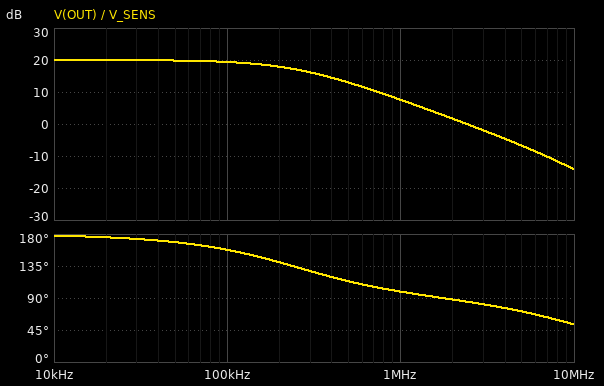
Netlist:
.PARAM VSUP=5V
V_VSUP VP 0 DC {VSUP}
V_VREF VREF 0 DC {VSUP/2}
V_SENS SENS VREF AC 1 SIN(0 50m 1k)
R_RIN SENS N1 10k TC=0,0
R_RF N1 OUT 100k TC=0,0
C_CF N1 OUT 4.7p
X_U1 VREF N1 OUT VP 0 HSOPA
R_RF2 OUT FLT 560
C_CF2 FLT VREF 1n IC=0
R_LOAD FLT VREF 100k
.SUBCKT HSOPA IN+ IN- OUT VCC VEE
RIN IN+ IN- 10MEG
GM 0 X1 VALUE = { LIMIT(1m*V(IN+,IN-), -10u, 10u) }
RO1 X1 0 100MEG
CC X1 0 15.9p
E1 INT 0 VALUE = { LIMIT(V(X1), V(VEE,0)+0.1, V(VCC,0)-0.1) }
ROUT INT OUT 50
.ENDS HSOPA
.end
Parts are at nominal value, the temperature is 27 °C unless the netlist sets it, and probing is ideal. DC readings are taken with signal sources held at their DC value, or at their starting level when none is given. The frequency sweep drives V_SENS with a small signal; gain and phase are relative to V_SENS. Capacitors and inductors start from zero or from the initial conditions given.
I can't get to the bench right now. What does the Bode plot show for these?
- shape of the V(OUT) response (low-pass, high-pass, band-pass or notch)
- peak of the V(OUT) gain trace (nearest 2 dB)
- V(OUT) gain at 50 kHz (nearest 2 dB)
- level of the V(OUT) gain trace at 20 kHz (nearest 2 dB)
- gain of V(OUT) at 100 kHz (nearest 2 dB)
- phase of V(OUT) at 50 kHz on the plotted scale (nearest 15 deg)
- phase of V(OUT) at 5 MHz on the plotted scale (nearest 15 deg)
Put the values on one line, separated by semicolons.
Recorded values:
low-pass; 20 dB; 20 dB; 20 dB; 20 dB; 165 deg; 75 deg
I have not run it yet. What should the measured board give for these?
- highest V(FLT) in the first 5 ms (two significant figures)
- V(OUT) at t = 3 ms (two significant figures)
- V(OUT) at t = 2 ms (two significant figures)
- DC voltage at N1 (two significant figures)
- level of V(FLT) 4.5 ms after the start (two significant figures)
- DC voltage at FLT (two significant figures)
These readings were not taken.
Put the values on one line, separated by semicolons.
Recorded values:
3.0 V; 2.5 V; 2.5 V; 2.5 V; 2.5 V; 2.5 V
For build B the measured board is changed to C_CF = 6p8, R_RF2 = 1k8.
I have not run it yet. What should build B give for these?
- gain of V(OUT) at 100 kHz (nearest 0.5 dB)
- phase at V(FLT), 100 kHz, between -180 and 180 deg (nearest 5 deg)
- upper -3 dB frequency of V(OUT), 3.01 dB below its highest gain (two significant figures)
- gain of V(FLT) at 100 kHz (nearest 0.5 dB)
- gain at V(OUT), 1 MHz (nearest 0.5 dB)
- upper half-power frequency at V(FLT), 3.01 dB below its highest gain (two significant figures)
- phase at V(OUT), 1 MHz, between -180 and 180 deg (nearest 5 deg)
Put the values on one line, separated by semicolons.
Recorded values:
19.0 dB; 105 deg; 190 kHz; 15.5 dB; 5.5 dB; 76 kHz; 95 deg
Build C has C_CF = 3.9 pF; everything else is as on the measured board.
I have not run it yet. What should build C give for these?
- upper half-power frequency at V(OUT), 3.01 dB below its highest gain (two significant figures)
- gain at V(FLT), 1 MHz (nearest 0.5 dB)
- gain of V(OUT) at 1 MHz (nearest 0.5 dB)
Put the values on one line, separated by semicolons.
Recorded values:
290 kHz; -2.5 dB; 8.5 dB
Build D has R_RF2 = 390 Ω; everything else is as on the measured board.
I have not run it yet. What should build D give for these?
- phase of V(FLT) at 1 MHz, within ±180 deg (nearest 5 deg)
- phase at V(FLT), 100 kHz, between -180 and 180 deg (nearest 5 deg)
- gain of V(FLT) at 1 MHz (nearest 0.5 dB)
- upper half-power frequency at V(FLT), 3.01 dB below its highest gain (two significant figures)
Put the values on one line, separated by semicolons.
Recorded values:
30 deg; 145 deg; -1.0 dB; 200 kHz
